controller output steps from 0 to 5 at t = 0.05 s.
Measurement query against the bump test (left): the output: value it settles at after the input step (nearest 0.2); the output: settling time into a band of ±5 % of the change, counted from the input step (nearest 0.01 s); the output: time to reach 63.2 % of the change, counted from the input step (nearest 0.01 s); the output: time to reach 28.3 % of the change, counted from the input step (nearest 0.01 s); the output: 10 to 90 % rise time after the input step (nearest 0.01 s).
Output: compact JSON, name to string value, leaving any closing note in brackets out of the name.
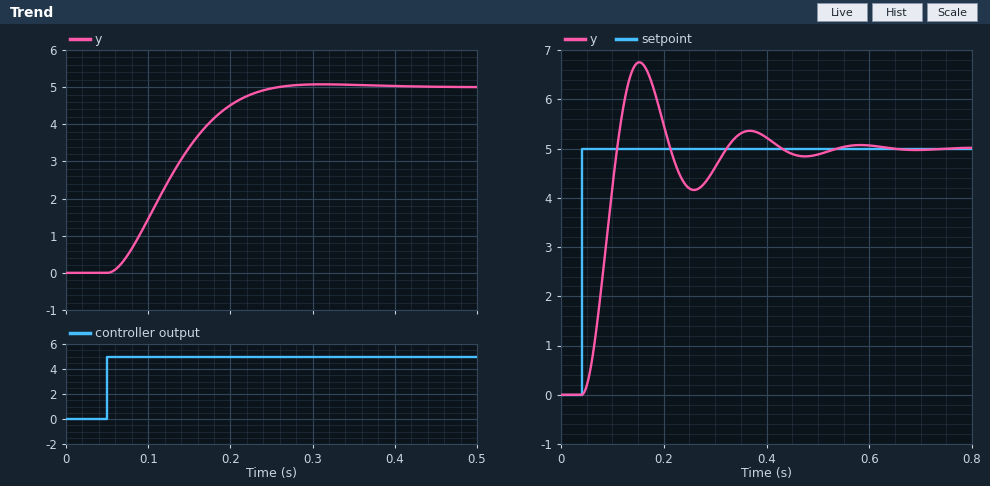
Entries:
{"the output: value it settles at after the input step": "5.0", "the output: settling time into a band of ±5 % of the change, counted from the input step": "0.17 s", "the output: time to reach 63.2 % of the change, counted from the input step": "0.09 s", "the output: time to reach 28.3 % of the change, counted from the input step": "0.05 s", "the output: 10 to 90 % rise time after the input step": "0.12 s"}
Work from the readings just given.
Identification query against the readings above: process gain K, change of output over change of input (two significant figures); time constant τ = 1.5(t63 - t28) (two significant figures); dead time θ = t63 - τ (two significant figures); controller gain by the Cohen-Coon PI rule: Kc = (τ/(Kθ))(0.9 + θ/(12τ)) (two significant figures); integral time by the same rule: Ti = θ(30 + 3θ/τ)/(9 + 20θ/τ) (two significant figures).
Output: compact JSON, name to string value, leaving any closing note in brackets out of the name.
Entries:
{"process gain K, change of output over change of input": "1.0", "time constant τ = 1.5(t63 - t28)": "0.060 s", "dead time θ = t63 - τ": "0.030 s", "controller gain by the Cohen-Coon PI rule: Kc = (τ/(Kθ))(0.9 + θ/(12τ))": "1.9", "integral time by the same rule: Ti = θ(30 + 3θ/τ)/(9 + 20θ/τ)": "0.050 s"}
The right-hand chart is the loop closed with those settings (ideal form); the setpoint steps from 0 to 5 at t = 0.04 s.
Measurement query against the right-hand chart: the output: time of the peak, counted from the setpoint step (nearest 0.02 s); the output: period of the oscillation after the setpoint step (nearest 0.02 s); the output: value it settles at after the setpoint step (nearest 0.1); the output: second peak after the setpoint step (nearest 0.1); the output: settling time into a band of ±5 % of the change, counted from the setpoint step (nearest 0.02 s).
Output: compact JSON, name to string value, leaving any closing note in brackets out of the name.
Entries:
{"the output: time of the peak, counted from the setpoint step": "0.12 s", "the output: period of the oscillation after the setpoint step": "0.22 s", "the output: value it settles at after the setpoint step": "5.0", "the output: second peak after the setpoint step": "5.4", "the output: settling time into a band of ±5 % of the change, counted from the setpoint step": "0.36 s"}
